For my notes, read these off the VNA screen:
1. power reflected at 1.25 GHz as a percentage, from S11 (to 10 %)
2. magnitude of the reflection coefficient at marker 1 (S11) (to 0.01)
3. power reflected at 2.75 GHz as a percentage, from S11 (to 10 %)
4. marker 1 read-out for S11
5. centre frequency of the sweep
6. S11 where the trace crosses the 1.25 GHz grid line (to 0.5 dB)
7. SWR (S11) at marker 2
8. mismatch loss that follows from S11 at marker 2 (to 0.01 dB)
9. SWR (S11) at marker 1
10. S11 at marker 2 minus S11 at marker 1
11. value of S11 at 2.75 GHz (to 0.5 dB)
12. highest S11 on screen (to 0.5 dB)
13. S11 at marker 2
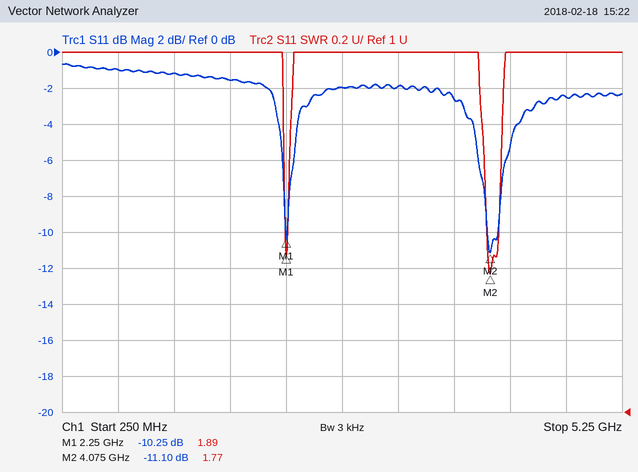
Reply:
80 %
0.31
60 %
-10.25 dB
2.75 GHz
-1.0 dB
1.77
0.35 dB
1.89
-0.85 dB
-2.0 dB
-0.5 dB
-11.10 dB
